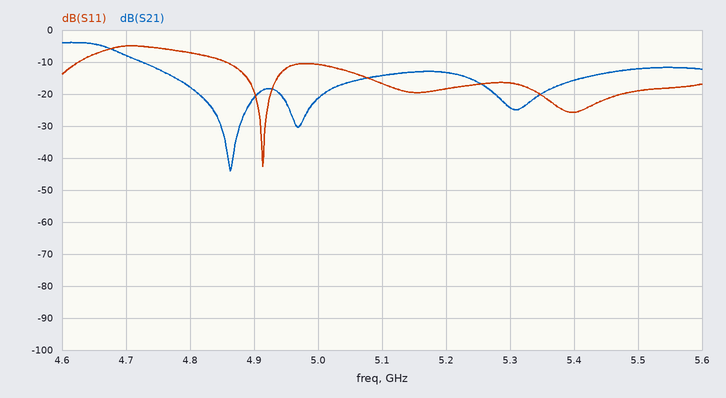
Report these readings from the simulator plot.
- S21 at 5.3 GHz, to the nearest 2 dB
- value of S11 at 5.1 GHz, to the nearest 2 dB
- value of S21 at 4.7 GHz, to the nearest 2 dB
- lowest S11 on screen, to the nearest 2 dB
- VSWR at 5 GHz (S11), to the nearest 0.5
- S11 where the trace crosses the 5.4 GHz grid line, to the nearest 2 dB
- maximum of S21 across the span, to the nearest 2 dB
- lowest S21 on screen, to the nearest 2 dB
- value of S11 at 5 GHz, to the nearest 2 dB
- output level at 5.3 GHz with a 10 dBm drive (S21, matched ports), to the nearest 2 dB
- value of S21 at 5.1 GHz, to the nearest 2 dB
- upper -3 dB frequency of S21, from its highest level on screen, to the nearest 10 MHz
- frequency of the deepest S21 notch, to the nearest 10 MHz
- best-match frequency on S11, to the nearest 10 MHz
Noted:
-24 dB
-16 dB
-8 dB
-42 dB
2.0
-26 dB
-4 dB
-44 dB
-10 dB
-14 dBm
-14 dB
4.69 GHz
4.86 GHz
4.91 GHz
